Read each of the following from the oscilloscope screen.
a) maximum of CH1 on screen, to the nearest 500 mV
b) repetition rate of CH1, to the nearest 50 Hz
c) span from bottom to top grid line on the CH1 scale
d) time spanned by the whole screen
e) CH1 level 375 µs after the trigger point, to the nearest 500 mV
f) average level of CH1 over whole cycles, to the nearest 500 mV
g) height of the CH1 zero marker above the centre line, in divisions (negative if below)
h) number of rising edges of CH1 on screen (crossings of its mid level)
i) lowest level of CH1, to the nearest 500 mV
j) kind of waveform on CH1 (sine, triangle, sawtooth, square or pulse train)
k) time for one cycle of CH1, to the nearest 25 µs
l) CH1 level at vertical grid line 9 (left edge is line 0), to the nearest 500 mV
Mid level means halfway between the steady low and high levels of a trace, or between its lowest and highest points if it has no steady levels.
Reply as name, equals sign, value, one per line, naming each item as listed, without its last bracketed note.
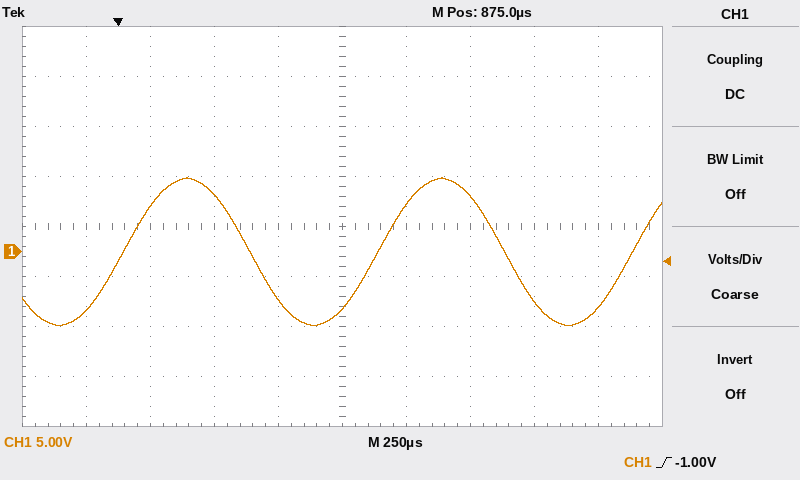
maximum of CH1 on screen, to the nearest 500 mV = 7.5 V
repetition rate of CH1, to the nearest 50 Hz = 1.00 kHz
span from bottom to top grid line on the CH1 scale = 40 V
time spanned by the whole screen = 2.5 ms
CH1 level 375 µs after the trigger point, to the nearest 500 mV = 5.5 V
average level of CH1 over whole cycles, to the nearest 500 mV = 0.0 V
height of the CH1 zero marker above the centre line, in divisions = -0.5 div
number of rising edges of CH1 on screen = 3
lowest level of CH1, to the nearest 500 mV = -7.5 V
kind of waveform on CH1 = sine
time for one cycle of CH1, to the nearest 25 µs = 1.000 ms
CH1 level at vertical grid line 9 (left edge is line 0), to the nearest 500 mV = -5.5 V
